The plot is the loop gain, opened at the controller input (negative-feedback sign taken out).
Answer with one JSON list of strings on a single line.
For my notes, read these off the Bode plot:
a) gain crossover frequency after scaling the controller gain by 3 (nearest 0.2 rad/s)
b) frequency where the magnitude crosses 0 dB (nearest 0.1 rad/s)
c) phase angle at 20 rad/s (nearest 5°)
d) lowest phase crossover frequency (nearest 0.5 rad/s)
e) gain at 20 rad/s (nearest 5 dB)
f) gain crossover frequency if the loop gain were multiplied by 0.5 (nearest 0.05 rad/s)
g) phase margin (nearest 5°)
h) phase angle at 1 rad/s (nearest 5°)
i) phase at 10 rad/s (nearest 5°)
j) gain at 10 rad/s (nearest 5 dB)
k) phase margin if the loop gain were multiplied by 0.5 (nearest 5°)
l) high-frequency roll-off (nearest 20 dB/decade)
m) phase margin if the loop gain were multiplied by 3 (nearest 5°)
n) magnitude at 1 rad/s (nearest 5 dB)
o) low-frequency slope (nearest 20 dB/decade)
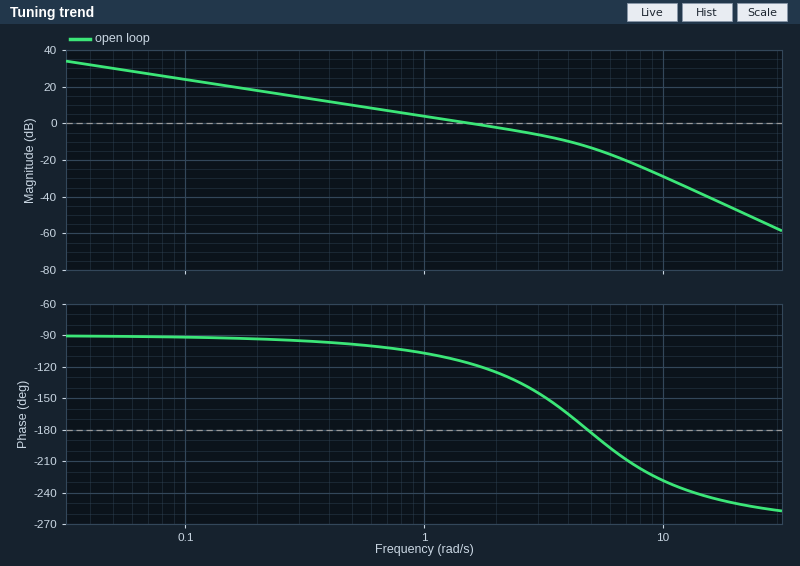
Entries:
["4.0 rad/s", "1.6 rad/s", "-250°", "5.0 rad/s", "-45 dB", "0.80 rad/s", "65°", "-105°", "-230°", "-30 dB", "75°", "-60 dB/decade", "15°", "5 dB", "-20 dB/decade"]
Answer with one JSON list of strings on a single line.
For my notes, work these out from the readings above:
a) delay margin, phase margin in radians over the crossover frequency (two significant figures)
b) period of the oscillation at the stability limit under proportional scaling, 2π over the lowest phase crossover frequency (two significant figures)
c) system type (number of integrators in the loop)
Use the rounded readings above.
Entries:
["0.71 s", "1.3 s", "1"]
